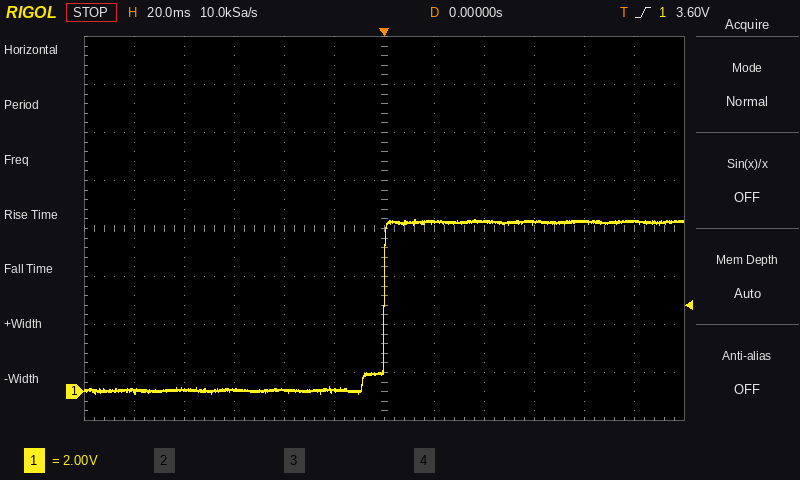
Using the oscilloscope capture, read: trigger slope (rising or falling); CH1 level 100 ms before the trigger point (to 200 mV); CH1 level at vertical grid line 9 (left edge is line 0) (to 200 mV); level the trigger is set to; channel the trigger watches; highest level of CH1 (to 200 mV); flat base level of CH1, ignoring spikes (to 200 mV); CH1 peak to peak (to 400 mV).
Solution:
rising
0.0 V
7.0 V
3.60 V
CH1
7.2 V
0.0 V
7.2 V
